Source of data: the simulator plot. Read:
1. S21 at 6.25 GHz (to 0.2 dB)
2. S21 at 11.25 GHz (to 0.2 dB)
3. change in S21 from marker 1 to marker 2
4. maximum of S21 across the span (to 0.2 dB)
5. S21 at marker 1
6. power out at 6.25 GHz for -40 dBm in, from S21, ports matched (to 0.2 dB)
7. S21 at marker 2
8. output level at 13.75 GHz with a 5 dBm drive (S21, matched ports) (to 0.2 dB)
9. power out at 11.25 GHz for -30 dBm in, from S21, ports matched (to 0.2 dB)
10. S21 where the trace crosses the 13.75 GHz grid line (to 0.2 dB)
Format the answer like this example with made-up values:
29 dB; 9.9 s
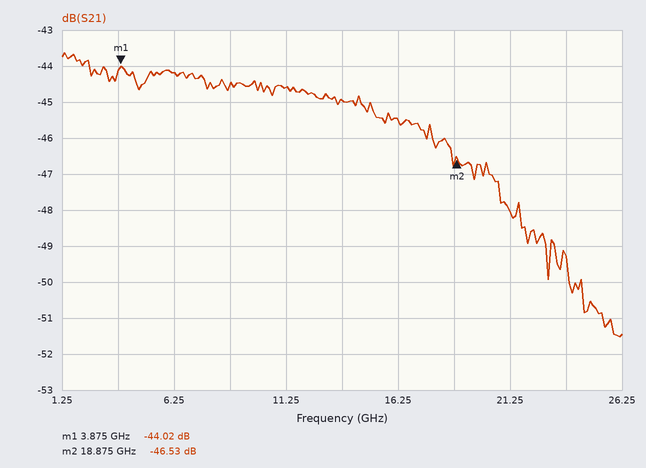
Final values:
-44.2 dB; -44.6 dB; -2.51 dB; -43.6 dB; -44.02 dB; -84.2 dBm; -46.53 dB; -40.0 dBm; -74.6 dBm; -45.0 dB
